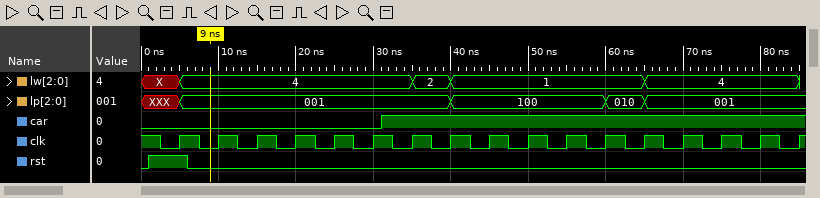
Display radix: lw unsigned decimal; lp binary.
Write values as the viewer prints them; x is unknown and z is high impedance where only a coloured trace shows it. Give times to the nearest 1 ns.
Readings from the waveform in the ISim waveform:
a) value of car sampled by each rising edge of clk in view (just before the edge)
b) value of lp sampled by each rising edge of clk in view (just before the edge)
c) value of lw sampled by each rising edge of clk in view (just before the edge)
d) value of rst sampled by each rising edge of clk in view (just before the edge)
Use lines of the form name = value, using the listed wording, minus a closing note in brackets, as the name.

value of car sampled by each rising edge of clk in view = 0 0 0 0 0 0 1 1 1 1 1 1 1 1 1 1 1
value of lp sampled by each rising edge of clk in view = XXX, 001, 001, 001, 001, 001, 001, 001, 100, 100, 100, 100, 010, 001, 001, 001, 001
value of lw sampled by each rising edge of clk in view = X, 4, 4, 4, 4, 4, 4, 2, 1, 1, 1, 1, 1, 4, 4, 4, 4
value of rst sampled by each rising edge of clk in view = 1 0 0 0 0 0 0 0 0 0 0 0 0 0 0 0 0
